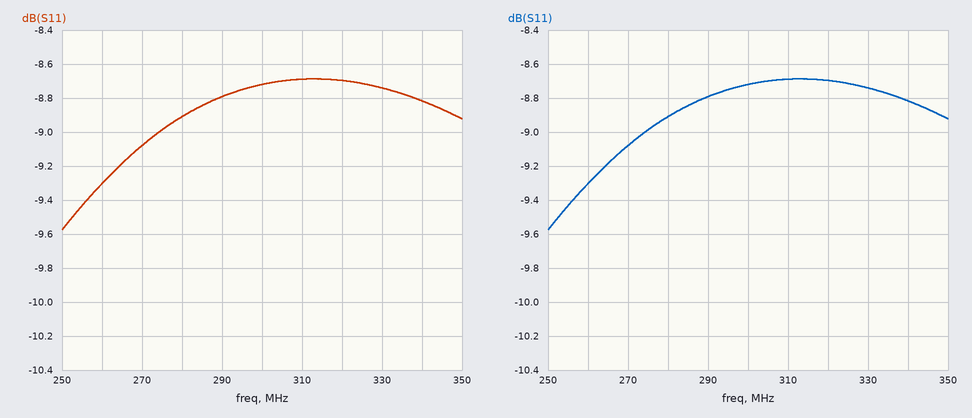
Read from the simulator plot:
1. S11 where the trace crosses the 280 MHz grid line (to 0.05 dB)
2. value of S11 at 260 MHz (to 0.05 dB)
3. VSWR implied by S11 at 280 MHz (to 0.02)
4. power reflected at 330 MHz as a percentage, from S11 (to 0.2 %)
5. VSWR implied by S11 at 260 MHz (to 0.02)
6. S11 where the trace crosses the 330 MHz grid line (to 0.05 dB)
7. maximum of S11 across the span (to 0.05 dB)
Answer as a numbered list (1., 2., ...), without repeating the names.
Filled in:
1. -8.90 dB
2. -9.30 dB
3. 2.12
4. 13.4 %
5. 2.04
6. -8.75 dB
7. -8.70 dB
